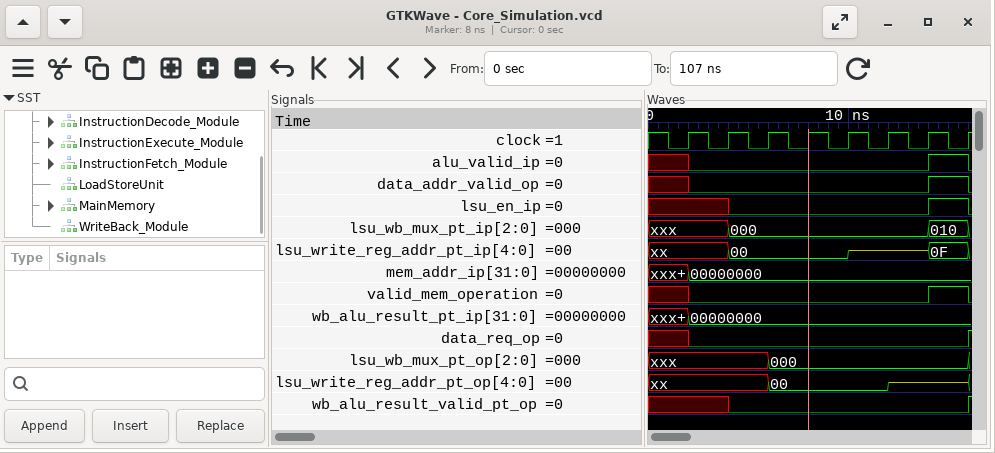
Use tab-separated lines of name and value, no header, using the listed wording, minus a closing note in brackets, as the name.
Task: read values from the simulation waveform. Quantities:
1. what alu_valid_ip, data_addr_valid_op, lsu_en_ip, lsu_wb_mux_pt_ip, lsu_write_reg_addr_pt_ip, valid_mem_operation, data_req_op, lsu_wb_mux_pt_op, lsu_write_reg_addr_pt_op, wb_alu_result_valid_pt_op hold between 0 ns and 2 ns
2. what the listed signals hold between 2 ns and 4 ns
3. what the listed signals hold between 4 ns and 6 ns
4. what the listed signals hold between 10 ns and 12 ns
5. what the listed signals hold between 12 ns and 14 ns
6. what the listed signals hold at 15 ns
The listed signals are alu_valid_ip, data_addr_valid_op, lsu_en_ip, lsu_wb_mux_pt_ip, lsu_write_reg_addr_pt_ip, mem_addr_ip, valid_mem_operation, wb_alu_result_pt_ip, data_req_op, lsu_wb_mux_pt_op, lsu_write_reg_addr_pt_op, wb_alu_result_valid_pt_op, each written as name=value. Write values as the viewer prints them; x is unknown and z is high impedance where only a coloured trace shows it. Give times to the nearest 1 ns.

what alu_valid_ip, data_addr_valid_op, lsu_en_ip, lsu_wb_mux_pt_ip, lsu_write_reg_addr_pt_ip, valid_mem_operation, data_req_op, lsu_wb_mux_pt_op, lsu_write_reg_addr_pt_op, wb_alu_result_valid_pt_op hold between 0 ns and 2 ns	alu_valid_ip=x, data_addr_valid_op=x, lsu_en_ip=x, lsu_wb_mux_pt_ip=xxx, lsu_write_reg_addr_pt_ip=xx, valid_mem_operation=x, data_req_op=x, lsu_wb_mux_pt_op=xxx, lsu_write_reg_addr_pt_op=xx, wb_alu_result_valid_pt_op=x
what the listed signals hold between 2 ns and 4 ns	alu_valid_ip=0, data_addr_valid_op=0, lsu_en_ip=x, lsu_wb_mux_pt_ip=xxx, lsu_write_reg_addr_pt_ip=xx, mem_addr_ip=00000000, valid_mem_operation=0, wb_alu_result_pt_ip=00000000, data_req_op=0, lsu_wb_mux_pt_op=xxx, lsu_write_reg_addr_pt_op=xx, wb_alu_result_valid_pt_op=x
what the listed signals hold between 4 ns and 6 ns	alu_valid_ip=0, data_addr_valid_op=0, lsu_en_ip=0, lsu_wb_mux_pt_ip=000, lsu_write_reg_addr_pt_ip=00, mem_addr_ip=00000000, valid_mem_operation=0, wb_alu_result_pt_ip=00000000, data_req_op=0, lsu_wb_mux_pt_op=xxx, lsu_write_reg_addr_pt_op=xx, wb_alu_result_valid_pt_op=0
what the listed signals hold between 10 ns and 12 ns	alu_valid_ip=0, data_addr_valid_op=0, lsu_en_ip=0, lsu_wb_mux_pt_ip=000, lsu_write_reg_addr_pt_ip=z, mem_addr_ip=00000000, valid_mem_operation=0, wb_alu_result_pt_ip=00000000, data_req_op=0, lsu_wb_mux_pt_op=000, lsu_write_reg_addr_pt_op=00, wb_alu_result_valid_pt_op=0
what the listed signals hold between 12 ns and 14 ns	alu_valid_ip=0, data_addr_valid_op=0, lsu_en_ip=0, lsu_wb_mux_pt_ip=000, lsu_write_reg_addr_pt_ip=z, mem_addr_ip=00000000, valid_mem_operation=0, wb_alu_result_pt_ip=00000000, data_req_op=0, lsu_wb_mux_pt_op=000, lsu_write_reg_addr_pt_op=z, wb_alu_result_valid_pt_op=0
what the listed signals hold at 15 ns	alu_valid_ip=1, data_addr_valid_op=1, lsu_en_ip=1, lsu_wb_mux_pt_ip=010, lsu_write_reg_addr_pt_ip=0F, mem_addr_ip=00000000, valid_mem_operation=1, wb_alu_result_pt_ip=00000000, data_req_op=0, lsu_wb_mux_pt_op=000, lsu_write_reg_addr_pt_op=z, wb_alu_result_valid_pt_op=0
